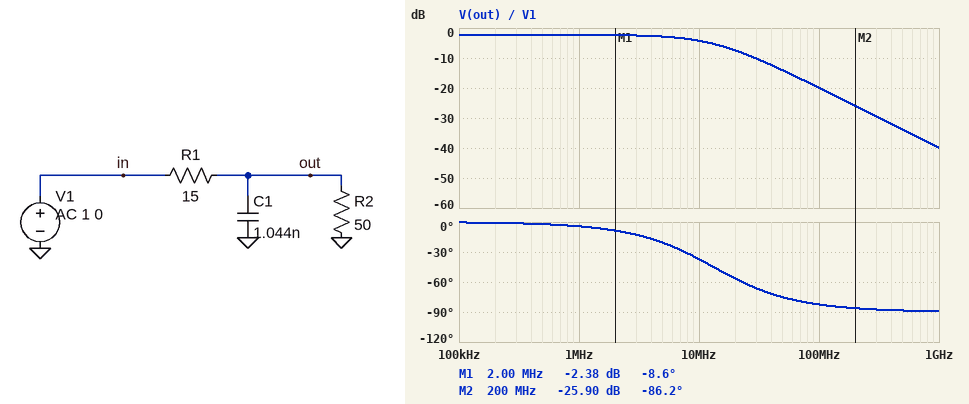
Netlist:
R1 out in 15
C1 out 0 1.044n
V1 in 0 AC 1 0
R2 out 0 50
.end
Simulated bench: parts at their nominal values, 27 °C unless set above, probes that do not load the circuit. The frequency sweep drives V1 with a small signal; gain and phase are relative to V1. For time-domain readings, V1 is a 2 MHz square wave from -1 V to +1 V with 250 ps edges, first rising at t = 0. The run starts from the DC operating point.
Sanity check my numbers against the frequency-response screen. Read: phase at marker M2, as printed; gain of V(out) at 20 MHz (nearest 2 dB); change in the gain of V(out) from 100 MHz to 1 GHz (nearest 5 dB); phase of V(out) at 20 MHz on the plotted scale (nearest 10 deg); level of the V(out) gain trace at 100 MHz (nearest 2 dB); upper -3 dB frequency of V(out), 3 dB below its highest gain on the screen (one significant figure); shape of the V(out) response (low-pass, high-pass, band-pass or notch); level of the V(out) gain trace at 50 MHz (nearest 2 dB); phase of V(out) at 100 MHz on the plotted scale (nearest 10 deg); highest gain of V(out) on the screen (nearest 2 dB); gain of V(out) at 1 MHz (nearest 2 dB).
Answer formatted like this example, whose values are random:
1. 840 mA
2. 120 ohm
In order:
1. -86.2 deg
2. -8 dB
3. -20 dB
4. -60 deg
5. -20 dB
6. 10 MHz
7. low-pass
8. -14 dB
9. -80 deg
10. -2 dB
11. -2 dB
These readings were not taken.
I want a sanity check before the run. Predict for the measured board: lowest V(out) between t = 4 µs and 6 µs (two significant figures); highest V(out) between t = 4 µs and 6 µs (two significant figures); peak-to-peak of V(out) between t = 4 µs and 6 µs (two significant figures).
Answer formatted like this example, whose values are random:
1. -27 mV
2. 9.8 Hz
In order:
1. -770 mV
2. 770 mV
3. 1.5 V
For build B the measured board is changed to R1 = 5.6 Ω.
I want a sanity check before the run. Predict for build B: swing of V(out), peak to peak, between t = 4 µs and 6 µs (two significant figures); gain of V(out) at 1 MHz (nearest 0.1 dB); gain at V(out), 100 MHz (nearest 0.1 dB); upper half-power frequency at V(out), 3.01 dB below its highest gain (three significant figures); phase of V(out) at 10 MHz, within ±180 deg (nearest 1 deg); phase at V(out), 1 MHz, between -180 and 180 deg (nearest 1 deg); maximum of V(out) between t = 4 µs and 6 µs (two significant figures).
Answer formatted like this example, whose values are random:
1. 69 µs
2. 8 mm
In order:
1. 1.8 V
2. -0.9 dB
3. -11.7 dB
4. 30.3 MHz
5. -18 deg
6. -2 deg
7. 900 mV
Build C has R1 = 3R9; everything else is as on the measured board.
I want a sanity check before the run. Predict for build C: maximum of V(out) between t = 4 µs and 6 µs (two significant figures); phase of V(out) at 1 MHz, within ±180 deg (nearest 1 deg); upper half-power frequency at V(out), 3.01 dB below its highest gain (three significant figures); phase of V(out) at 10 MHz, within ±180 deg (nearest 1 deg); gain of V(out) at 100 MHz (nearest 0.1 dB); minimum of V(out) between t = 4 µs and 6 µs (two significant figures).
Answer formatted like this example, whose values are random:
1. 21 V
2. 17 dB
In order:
1. 930 mV
2. -1 deg
3. 42.1 MHz
4. -13 deg
5. -8.9 dB
6. -930 mV
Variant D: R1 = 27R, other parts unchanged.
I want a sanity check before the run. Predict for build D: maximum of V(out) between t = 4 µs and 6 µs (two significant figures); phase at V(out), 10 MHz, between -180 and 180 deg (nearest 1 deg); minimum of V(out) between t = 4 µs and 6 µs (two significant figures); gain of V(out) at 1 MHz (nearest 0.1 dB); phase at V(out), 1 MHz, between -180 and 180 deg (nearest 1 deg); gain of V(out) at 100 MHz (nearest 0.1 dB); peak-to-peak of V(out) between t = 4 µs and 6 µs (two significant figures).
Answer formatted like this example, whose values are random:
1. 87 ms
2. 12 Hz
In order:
1. 650 mV
2. -49 deg
3. -650 mV
4. -3.8 dB
5. -7 deg
6. -25.0 dB
7. 1.3 V
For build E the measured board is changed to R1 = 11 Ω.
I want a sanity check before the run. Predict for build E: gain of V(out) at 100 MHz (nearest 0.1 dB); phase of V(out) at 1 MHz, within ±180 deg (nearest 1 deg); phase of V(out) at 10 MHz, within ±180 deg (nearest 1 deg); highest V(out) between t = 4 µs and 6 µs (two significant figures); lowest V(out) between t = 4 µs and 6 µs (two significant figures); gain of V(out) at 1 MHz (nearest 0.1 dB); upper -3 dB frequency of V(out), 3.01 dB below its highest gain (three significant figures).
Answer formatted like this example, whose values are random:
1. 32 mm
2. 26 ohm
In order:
1. -17.3 dB
2. -3 deg
3. -31 deg
4. 820 mV
5. -820 mV
6. -1.7 dB
7. 16.9 MHz
